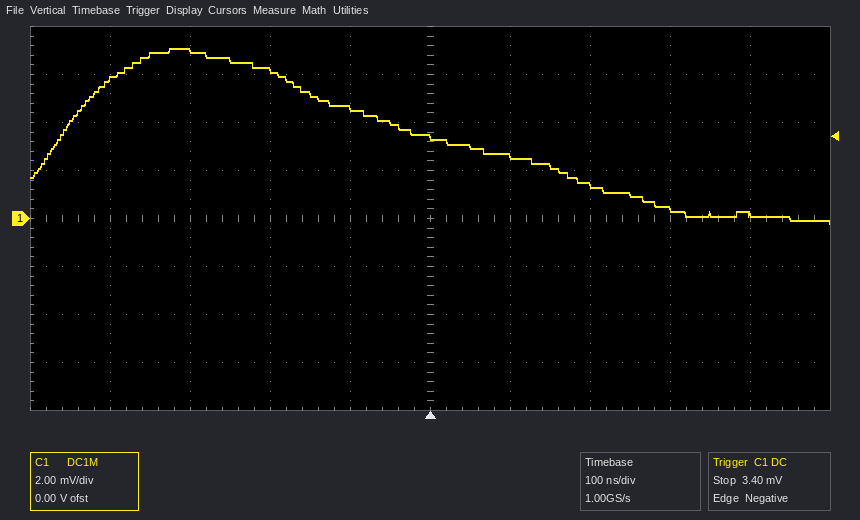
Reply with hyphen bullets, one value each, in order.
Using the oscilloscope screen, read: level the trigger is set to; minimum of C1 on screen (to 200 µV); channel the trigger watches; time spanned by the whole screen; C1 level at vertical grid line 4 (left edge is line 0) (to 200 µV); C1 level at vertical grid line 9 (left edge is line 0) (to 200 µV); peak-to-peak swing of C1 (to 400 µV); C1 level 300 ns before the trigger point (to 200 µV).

- 3.40 mV
- -200 µV
- C1
- 1 µs
- 4.6 mV
- 200 µV
- 7.2 mV
- 7.0 mV
